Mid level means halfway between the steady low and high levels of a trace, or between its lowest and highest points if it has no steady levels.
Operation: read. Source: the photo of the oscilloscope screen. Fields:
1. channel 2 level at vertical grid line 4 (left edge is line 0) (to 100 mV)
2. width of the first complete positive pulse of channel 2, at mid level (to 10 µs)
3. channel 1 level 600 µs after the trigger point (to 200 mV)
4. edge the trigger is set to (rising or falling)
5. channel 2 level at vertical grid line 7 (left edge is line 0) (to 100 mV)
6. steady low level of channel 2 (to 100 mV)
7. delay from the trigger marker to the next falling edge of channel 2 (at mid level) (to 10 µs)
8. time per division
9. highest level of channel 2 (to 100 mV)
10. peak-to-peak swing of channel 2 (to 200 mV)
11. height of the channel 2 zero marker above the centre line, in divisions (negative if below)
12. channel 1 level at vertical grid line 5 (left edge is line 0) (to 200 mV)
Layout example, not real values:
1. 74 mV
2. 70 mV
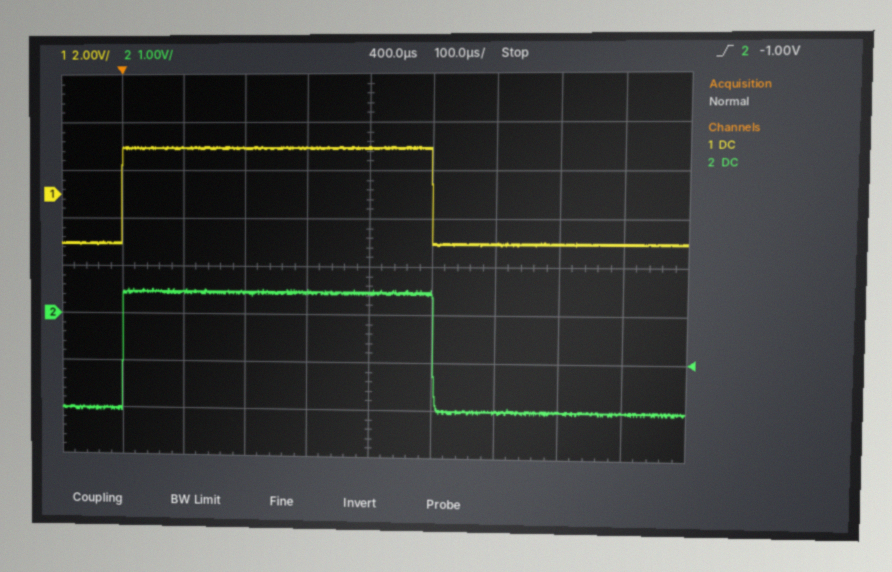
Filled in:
1. 500 mV
2. 500 µs
3. -2.0 V
4. rising
5. -2.0 V
6. -2.0 V
7. 500 µs
8. 100 µs
9. 500 mV
10. 2.6 V
11. -1.0 div
12. 2.0 V
